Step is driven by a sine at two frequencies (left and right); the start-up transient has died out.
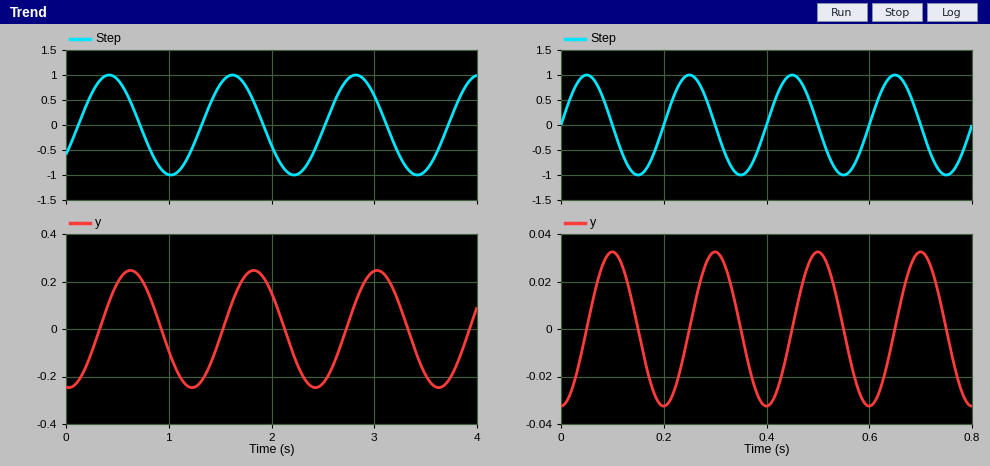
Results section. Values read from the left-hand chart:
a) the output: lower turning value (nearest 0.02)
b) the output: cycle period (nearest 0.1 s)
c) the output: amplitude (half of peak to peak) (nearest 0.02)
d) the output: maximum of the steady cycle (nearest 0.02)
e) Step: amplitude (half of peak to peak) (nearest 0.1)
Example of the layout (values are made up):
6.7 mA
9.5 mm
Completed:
-0.24
1.2 s
0.24
0.24
1.0
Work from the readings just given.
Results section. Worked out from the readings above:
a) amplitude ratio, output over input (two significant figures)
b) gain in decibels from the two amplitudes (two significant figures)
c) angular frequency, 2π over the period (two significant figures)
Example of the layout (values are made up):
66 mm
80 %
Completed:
0.24
-12 dB
5.2 rad/s
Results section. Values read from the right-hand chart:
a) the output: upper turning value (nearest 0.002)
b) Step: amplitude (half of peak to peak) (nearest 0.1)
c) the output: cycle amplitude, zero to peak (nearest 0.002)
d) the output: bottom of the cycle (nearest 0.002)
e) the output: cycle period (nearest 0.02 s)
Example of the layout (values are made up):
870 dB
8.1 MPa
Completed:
0.032
1.0
0.032
-0.032
0.20 s
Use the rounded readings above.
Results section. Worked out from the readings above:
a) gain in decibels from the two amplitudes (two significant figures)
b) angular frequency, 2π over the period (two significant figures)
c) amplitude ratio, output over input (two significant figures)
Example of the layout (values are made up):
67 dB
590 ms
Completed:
-30 dB
31 rad/s
0.032
